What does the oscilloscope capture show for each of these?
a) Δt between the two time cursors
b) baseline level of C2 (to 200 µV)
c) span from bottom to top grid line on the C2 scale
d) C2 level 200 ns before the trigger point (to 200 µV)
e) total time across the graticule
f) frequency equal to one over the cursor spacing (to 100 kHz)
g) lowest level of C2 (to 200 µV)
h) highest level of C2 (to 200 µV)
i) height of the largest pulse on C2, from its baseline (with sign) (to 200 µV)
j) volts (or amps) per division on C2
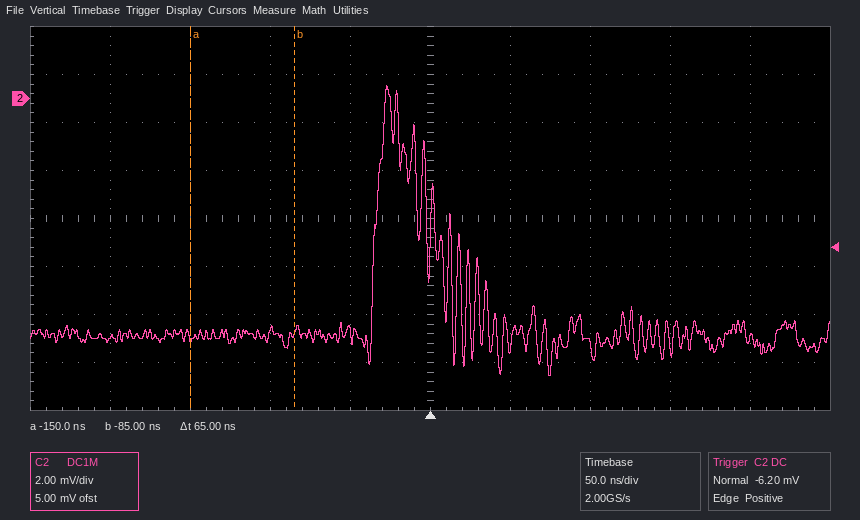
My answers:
65 ns
-9.8 mV
16 mV
-10.0 mV
500 ns
15.4 MHz
-11.6 mV
600 µV
+10.4 mV
2 mV
